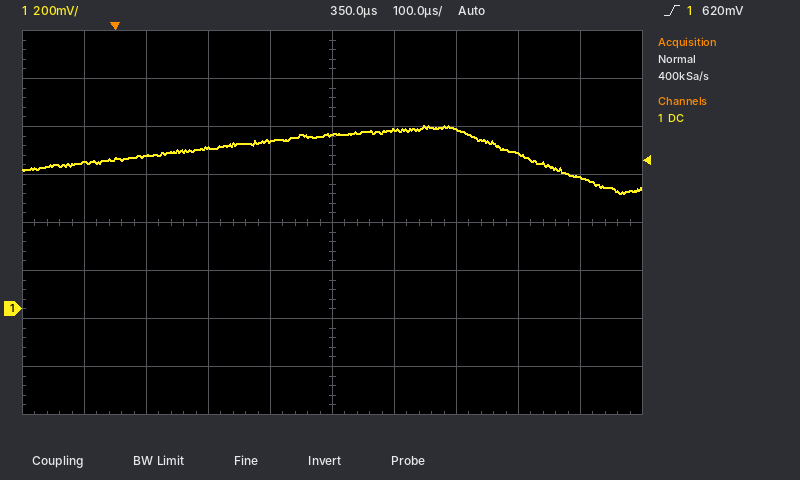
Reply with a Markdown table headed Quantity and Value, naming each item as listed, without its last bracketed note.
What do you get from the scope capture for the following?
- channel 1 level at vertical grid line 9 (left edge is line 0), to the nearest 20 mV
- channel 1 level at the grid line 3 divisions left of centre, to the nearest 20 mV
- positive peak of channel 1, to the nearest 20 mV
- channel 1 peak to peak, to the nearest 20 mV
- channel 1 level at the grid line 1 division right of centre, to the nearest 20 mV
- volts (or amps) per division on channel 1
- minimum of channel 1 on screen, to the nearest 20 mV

| Quantity | Value |
|---|---|
| channel 1 level at vertical grid line 9 (left edge is line 0), to the nearest 20 mV | 540 mV |
| channel 1 level at the grid line 3 divisions left of centre, to the nearest 20 mV | 640 mV |
| positive peak of channel 1, to the nearest 20 mV | 760 mV |
| channel 1 peak to peak, to the nearest 20 mV | 280 mV |
| channel 1 level at the grid line 1 division right of centre, to the nearest 20 mV | 740 mV |
| volts (or amps) per division on channel 1 | 200 mV |
| minimum of channel 1 on screen, to the nearest 20 mV | 480 mV |
